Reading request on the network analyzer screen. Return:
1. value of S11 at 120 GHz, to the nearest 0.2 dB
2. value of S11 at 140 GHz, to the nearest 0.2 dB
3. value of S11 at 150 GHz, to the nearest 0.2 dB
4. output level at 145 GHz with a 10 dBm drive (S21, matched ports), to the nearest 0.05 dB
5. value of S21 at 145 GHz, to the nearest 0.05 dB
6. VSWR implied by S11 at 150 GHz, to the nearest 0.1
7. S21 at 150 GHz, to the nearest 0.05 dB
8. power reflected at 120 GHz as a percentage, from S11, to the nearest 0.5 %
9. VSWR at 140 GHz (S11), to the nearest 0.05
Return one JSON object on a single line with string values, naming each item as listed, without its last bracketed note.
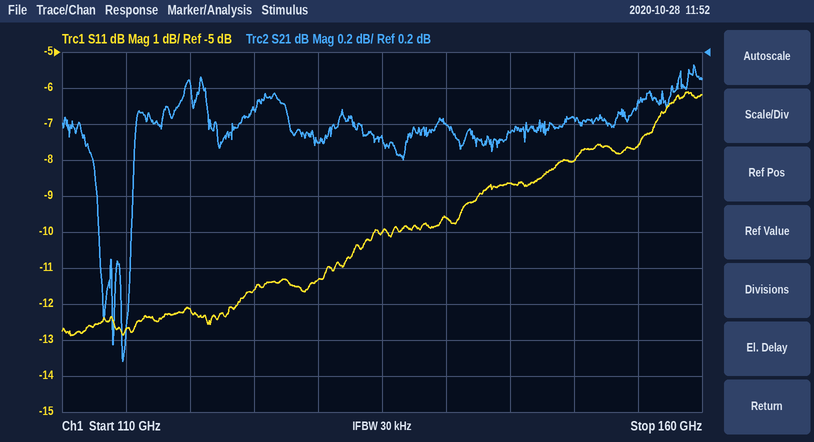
{"value of S11 at 120 GHz, to the nearest 0.2 dB": "-12.2 dB", "value of S11 at 140 GHz, to the nearest 0.2 dB": "-9.6 dB", "value of S11 at 150 GHz, to the nearest 0.2 dB": "-8.0 dB", "output level at 145 GHz with a 10 dBm drive (S21, matched ports), to the nearest 0.05 dB": "9.75 dBm", "value of S21 at 145 GHz, to the nearest 0.05 dB": "-0.25 dB", "VSWR implied by S11 at 150 GHz, to the nearest 0.1": "2.3", "S21 at 150 GHz, to the nearest 0.05 dB": "-0.15 dB", "power reflected at 120 GHz as a percentage, from S11, to the nearest 0.5 %": "6.0 %", "VSWR at 140 GHz (S11), to the nearest 0.05": "2.00"}
